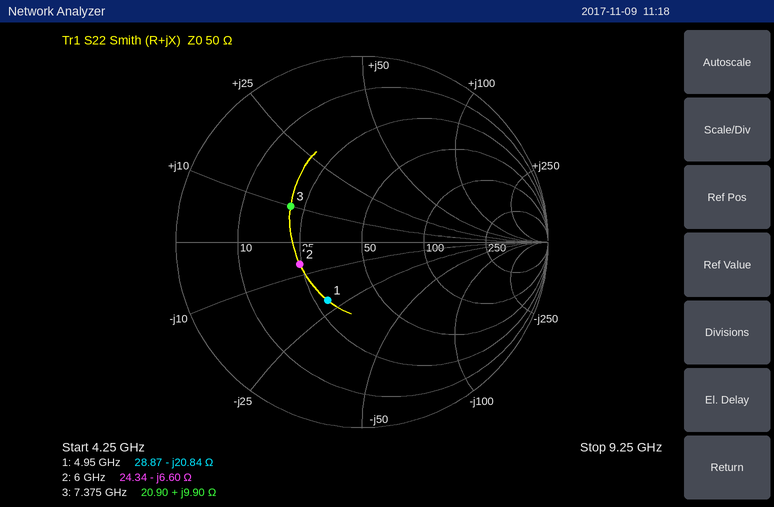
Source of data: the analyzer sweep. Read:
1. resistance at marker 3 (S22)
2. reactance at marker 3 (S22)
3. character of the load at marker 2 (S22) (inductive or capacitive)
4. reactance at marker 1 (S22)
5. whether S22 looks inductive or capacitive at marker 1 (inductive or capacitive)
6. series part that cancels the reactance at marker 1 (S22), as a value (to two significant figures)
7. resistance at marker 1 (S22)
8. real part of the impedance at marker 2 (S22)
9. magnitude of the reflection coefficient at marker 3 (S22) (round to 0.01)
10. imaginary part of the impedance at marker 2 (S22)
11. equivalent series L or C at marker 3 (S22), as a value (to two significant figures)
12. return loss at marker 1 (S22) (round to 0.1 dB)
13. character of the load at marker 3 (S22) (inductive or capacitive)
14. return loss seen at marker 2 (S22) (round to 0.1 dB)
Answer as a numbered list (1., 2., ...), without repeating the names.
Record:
1. 20.90 Ω
2. +9.90 Ω
3. capacitive
4. -20.84 Ω
5. capacitive
6. 670 pH
7. 28.87 Ω
8. 24.34 Ω
9. 0.43
10. -6.60 Ω
11. 210 pH
12. 8.8 dB
13. inductive
14. 9.0 dB
